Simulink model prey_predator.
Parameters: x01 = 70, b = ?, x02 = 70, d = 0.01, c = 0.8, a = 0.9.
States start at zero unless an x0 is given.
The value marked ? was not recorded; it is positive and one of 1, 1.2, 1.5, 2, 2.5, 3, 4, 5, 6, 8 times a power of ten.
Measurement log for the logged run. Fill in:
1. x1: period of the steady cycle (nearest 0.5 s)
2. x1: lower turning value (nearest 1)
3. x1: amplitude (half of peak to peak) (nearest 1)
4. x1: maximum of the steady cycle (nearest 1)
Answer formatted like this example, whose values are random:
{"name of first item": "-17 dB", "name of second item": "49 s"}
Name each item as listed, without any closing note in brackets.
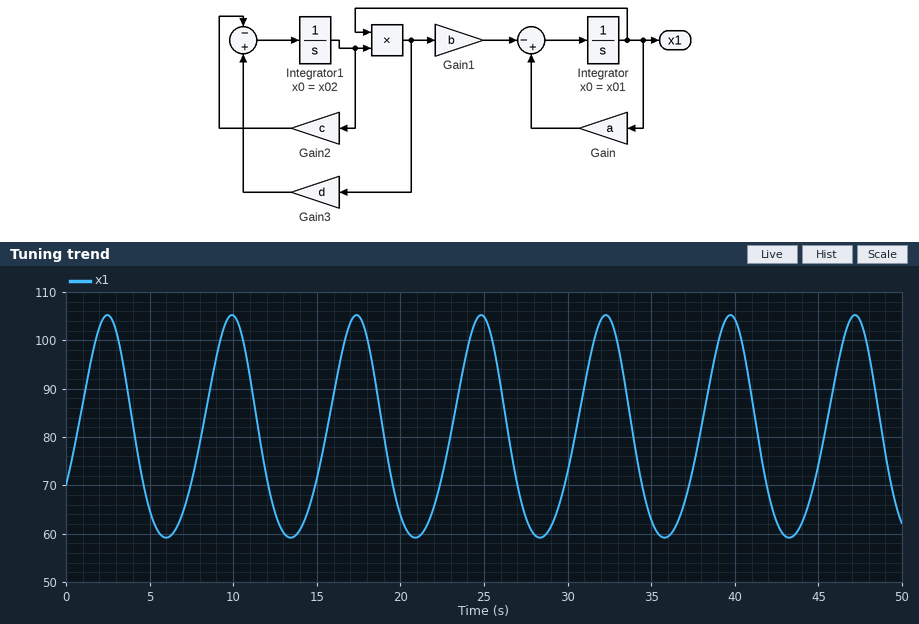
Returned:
{"x1: period of the steady cycle": "7.5 s", "x1: lower turning value": "59", "x1: amplitude (half of peak to peak)": "23", "x1: maximum of the steady cycle": "105"}
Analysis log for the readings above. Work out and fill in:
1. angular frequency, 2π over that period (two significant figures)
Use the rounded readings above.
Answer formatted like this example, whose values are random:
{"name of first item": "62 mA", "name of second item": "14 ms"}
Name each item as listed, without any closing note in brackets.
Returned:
{"angular frequency, 2π over that period": "0.84 rad/s"}
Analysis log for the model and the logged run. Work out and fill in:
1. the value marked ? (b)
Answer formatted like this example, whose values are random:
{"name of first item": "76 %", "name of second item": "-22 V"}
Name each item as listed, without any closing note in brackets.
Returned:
{"the value marked ?": "0.01"}
